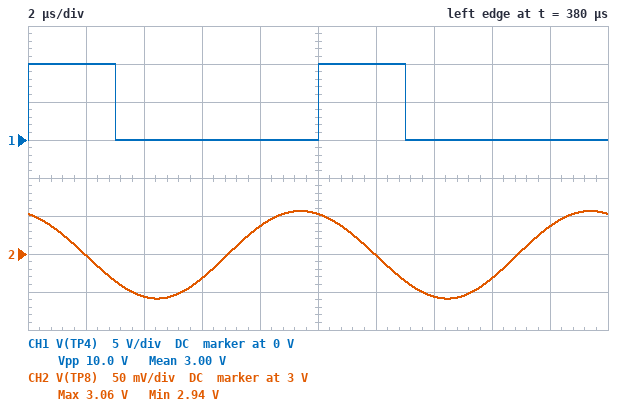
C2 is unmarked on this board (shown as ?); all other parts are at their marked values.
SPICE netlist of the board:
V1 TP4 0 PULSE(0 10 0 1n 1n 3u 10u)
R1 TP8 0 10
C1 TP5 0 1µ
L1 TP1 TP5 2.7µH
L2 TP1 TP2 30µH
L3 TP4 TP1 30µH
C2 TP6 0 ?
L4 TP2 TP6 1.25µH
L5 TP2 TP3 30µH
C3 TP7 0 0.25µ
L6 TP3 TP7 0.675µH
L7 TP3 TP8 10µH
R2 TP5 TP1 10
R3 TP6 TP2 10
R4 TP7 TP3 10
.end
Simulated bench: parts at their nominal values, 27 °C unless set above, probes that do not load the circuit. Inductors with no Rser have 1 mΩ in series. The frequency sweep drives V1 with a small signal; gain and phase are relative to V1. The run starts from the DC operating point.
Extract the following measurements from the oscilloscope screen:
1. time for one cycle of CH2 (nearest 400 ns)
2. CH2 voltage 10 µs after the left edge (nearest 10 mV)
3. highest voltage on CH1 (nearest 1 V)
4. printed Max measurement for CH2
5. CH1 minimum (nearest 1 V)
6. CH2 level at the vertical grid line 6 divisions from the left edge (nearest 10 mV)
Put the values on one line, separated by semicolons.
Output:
10.0 µs; 3.05 V; 10 V; 3.06 V; 0 V; 3.00 V
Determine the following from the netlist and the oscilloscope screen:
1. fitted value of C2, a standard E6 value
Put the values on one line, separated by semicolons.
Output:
150 nF
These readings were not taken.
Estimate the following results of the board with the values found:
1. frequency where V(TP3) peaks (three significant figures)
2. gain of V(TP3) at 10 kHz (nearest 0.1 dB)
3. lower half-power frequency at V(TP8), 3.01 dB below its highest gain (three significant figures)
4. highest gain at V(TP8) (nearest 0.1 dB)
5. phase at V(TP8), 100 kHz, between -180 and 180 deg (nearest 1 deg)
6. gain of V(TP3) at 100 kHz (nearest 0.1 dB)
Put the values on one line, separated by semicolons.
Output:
29.8 kHz; 0.5 dB; 21.8 kHz; 6.0 dB; 75 deg; -37.6 dB
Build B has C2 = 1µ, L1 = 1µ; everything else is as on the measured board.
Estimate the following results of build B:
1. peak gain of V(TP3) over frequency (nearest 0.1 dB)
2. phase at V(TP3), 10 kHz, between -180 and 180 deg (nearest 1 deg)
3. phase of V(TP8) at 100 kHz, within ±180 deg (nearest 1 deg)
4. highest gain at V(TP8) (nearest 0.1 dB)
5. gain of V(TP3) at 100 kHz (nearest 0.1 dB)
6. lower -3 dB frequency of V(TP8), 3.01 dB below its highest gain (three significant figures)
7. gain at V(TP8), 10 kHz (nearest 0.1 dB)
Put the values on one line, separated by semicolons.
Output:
5.3 dB; -38 deg; -158 deg; 5.2 dB; -56.8 dB; 10.0 kHz; 2.2 dB
